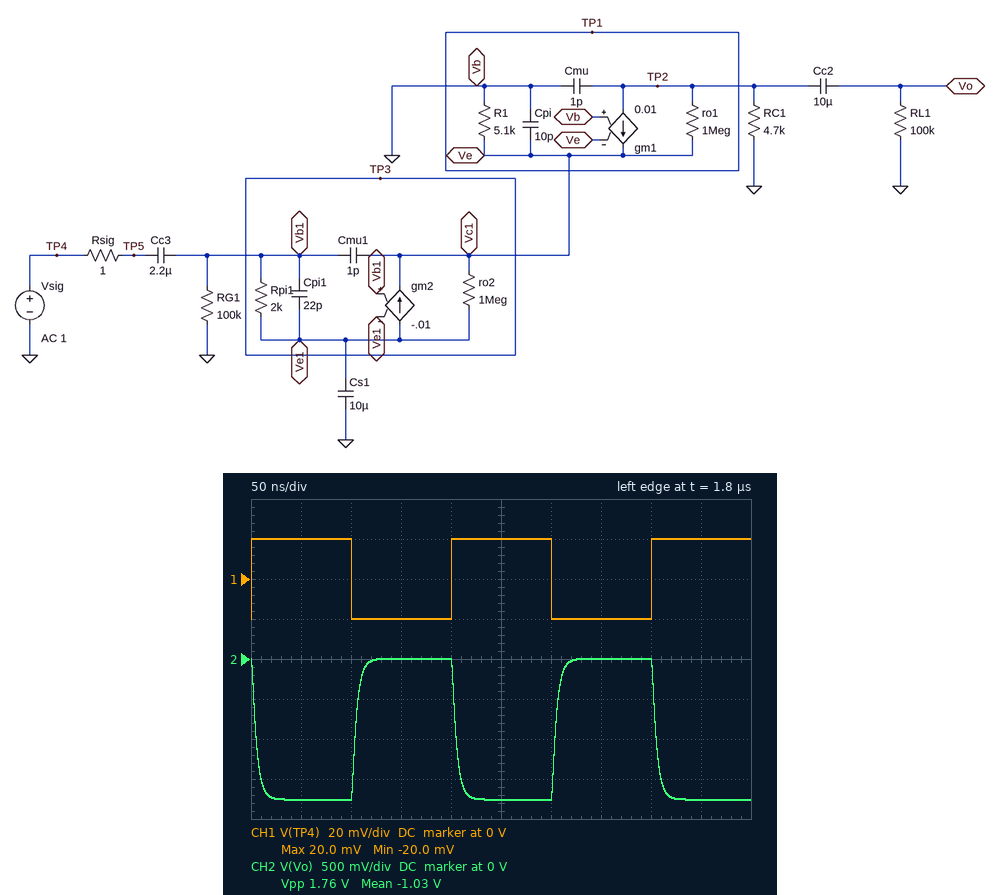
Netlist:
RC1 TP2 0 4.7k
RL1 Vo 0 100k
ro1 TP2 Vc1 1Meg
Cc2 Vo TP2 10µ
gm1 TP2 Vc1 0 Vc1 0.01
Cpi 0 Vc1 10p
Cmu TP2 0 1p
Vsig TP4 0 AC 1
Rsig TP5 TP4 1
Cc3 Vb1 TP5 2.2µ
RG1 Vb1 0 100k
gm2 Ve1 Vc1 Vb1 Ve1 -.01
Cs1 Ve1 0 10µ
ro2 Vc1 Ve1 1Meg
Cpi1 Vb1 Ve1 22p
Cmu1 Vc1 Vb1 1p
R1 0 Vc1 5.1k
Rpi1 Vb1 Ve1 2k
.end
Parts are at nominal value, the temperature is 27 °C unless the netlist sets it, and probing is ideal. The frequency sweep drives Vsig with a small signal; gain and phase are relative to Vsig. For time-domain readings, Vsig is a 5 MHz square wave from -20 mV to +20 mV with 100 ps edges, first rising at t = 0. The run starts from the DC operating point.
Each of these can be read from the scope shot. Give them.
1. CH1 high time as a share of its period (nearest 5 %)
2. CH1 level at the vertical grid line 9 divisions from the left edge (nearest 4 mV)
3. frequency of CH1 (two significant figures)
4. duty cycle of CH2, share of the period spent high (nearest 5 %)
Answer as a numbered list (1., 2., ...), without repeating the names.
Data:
1. 50 %
2. 20 mV
3. 5.0 MHz
4. 50 %
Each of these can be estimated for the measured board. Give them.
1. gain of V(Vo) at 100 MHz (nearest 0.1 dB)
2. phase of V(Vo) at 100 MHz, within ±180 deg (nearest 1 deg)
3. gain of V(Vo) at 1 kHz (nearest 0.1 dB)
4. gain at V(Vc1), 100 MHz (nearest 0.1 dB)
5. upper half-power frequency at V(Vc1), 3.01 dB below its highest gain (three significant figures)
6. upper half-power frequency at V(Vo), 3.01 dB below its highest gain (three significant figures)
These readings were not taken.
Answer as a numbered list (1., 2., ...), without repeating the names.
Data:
1. 21.7 dB
2. 71 deg
3. 32.7 dB
4. -1.8 dB
5. 147 MHz
6. 33.6 MHz
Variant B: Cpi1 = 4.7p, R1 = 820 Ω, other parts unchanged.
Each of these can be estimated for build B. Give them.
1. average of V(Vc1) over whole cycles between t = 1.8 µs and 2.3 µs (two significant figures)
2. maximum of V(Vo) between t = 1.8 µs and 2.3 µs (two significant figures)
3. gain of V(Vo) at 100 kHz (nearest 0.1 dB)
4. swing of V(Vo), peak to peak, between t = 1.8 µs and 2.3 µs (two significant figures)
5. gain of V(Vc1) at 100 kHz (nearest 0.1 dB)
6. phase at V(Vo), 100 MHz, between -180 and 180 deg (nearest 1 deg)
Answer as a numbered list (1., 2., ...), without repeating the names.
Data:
1. -18 mV
2. 3.7 mV
3. 32.0 dB
4. 1.6 V
5. -1.0 dB
6. 74 deg
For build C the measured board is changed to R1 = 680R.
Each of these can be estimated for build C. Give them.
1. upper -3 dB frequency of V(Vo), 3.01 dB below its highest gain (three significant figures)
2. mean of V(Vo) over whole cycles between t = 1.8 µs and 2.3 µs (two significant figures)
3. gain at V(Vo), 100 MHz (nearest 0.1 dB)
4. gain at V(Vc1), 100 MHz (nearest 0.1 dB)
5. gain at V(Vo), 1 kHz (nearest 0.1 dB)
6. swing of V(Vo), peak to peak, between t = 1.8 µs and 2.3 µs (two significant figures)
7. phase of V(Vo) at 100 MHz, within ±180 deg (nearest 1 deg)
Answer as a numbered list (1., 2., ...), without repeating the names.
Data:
1. 34.0 MHz
2. -780 mV
3. 21.0 dB
4. -2.5 dB
5. 31.7 dB
6. 1.6 V
7. 74 deg
